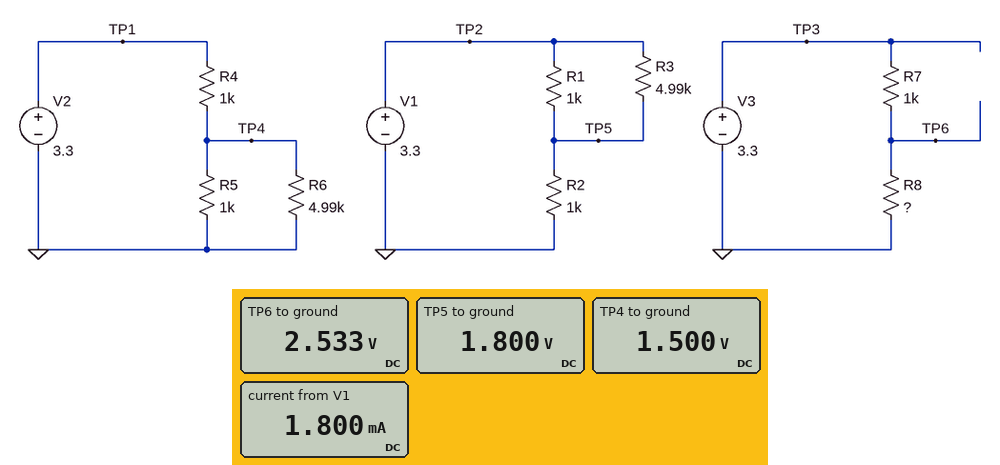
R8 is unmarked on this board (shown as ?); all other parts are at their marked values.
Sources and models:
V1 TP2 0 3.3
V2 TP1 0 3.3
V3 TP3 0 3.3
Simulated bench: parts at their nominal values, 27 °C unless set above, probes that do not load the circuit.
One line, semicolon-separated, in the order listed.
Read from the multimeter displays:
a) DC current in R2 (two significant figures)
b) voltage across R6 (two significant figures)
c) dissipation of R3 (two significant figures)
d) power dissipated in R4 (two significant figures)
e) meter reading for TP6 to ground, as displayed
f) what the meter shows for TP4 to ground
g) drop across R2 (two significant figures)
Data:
1.8 mA; 1.5 V; 450 µW; 3.2 mW; 2.533 V; 1.500 V; 1.8 V
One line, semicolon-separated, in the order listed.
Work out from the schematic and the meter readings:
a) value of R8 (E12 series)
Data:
3.3 kΩ
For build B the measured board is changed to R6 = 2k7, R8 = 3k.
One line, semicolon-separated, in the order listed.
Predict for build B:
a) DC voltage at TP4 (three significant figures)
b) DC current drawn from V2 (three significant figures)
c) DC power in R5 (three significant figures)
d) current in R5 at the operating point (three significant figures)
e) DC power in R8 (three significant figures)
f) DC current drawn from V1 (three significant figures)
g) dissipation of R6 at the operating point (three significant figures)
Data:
1.39 V; 1.91 mA; 1.94 mW; 1.39 mA; 2.04 mW; 1.80 mA; 718 µW
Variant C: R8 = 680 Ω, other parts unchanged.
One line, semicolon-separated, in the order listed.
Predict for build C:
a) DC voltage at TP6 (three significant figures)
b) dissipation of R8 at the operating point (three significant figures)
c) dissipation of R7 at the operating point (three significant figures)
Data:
1.34 V; 2.62 mW; 3.86 mW
